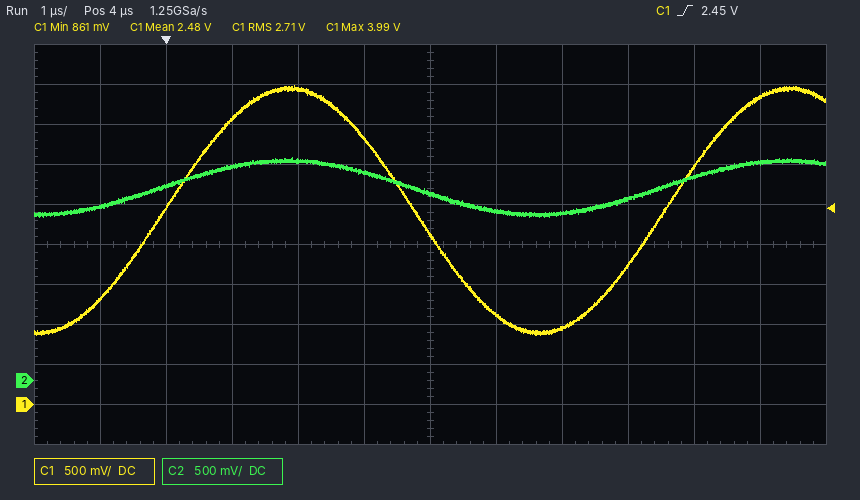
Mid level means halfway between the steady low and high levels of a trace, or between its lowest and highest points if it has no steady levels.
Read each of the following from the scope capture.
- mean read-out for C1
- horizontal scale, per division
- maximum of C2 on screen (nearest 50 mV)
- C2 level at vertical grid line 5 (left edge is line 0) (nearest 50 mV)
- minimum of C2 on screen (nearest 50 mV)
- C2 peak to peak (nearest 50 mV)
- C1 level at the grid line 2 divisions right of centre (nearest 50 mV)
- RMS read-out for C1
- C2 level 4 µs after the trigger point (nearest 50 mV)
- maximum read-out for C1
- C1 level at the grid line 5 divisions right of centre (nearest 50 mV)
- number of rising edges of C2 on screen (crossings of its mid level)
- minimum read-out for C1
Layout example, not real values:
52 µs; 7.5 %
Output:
2.48 V; 1 µs; 2.80 V; 2.60 V; 2.05 V; 750 mV; 950 mV; 2.71 V; 2.35 V; 3.99 V; 3.85 V; 2; 861 mV
